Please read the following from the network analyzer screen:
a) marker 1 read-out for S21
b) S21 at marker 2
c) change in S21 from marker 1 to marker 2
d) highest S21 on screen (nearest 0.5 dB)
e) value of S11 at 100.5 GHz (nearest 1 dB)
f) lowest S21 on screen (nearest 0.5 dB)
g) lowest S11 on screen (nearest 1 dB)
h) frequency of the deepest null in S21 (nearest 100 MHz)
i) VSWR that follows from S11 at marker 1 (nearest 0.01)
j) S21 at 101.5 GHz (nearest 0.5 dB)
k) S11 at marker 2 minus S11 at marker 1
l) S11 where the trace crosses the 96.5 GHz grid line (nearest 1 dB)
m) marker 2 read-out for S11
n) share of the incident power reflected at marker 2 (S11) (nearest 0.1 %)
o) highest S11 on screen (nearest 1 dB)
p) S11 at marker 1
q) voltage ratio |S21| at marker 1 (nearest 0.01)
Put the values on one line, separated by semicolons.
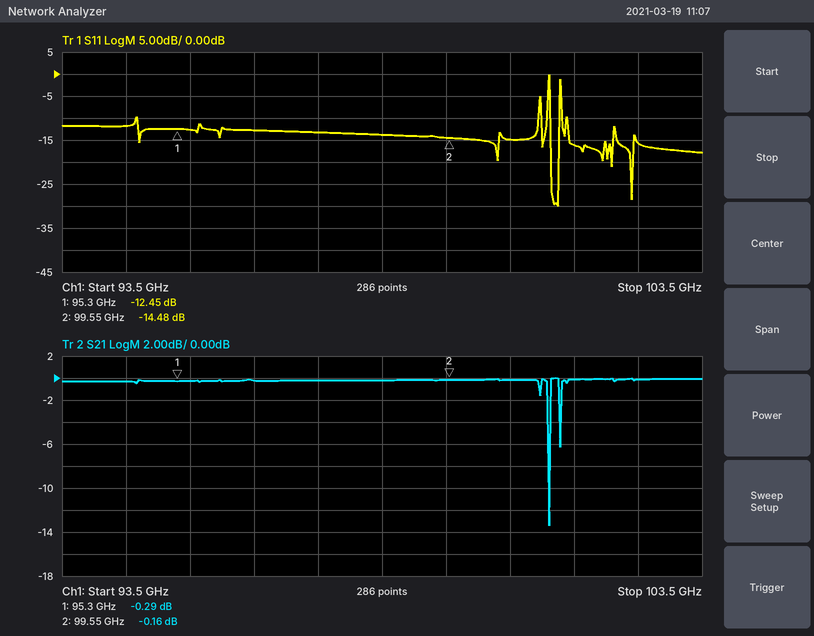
-0.29 dB; -0.16 dB; 0.13 dB; 0.0 dB; -15 dB; -13.5 dB; -30 dB; 101.1 GHz; 1.63; 0.0 dB; -2.03 dB; -13 dB; -14.48 dB; 3.6 %; 0 dB; -12.45 dB; 0.97
